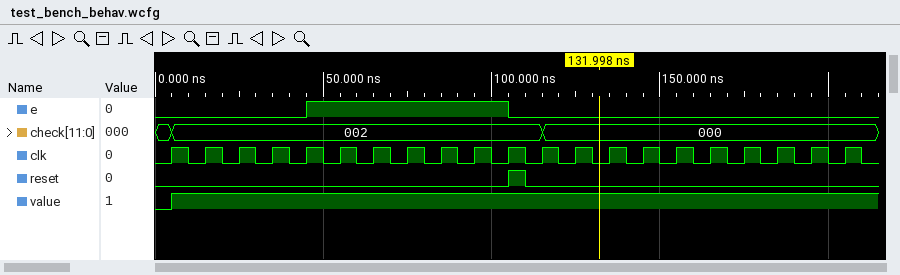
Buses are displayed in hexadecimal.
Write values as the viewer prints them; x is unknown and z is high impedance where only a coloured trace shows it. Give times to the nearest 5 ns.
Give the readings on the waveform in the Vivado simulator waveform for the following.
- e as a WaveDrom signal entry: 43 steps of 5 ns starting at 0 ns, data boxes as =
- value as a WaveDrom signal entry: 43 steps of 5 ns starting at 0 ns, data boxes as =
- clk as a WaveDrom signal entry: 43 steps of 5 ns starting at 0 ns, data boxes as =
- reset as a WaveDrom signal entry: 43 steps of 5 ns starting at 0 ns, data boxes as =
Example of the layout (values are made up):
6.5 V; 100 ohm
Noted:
{name: 'e', wave: '0........1...........0.....................'}; {name: 'value', wave: '01.........................................'}; {name: 'clk', wave: '0101010101010101010101010101010101010101010'}; {name: 'reset', wave: '0....................10....................'}
